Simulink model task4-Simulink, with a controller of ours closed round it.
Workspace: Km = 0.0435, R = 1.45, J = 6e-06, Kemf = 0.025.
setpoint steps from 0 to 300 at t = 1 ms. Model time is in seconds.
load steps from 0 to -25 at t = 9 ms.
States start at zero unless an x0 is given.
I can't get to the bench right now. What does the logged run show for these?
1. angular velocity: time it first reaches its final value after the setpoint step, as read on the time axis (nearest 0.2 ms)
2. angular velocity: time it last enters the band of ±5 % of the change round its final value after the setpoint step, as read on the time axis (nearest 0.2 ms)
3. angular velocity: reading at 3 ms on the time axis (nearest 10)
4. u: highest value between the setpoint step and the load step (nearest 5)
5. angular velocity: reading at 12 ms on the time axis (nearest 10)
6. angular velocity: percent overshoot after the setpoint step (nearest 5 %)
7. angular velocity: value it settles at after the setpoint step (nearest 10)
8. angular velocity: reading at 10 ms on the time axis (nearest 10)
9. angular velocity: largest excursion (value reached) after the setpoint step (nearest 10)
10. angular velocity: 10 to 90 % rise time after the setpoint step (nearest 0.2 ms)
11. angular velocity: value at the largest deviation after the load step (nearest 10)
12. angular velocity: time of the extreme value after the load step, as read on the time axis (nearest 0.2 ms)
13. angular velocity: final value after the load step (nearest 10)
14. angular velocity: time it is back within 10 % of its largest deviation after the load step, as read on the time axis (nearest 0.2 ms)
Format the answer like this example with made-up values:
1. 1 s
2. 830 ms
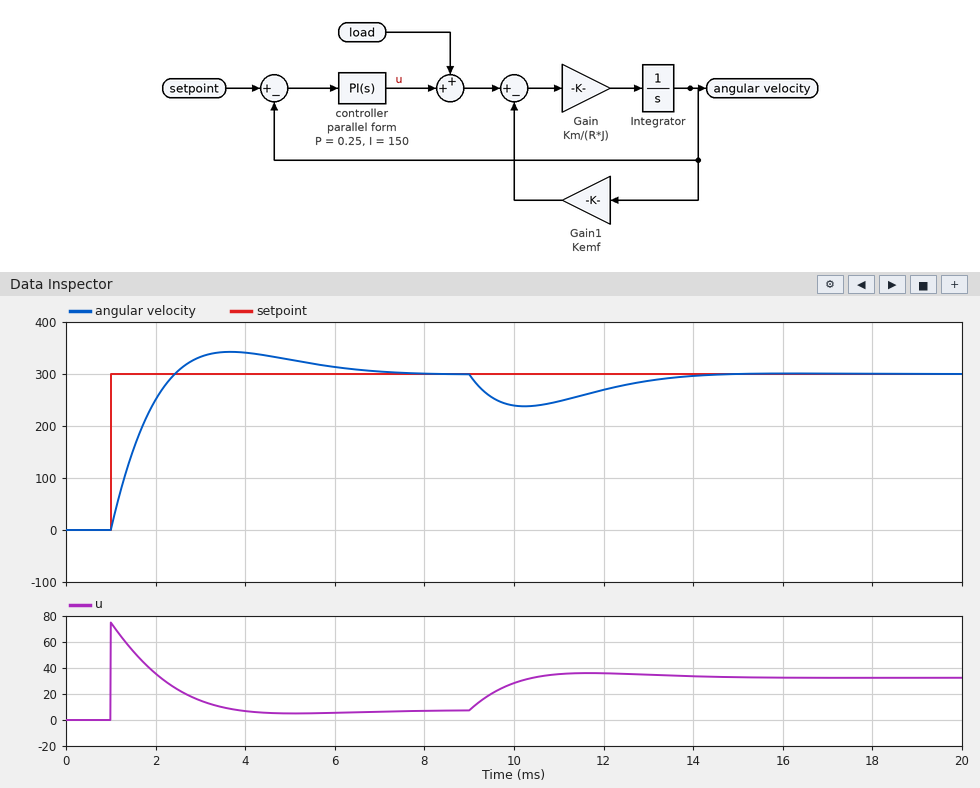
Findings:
1. 2.4 ms
2. 5.8 ms
3. 330
4. 75
5. 270
6. 15 %
7. 300
8. 240
9. 340
10. 1.0 ms
11. 240
12. 10.2 ms
13. 300
14. 13.6 ms
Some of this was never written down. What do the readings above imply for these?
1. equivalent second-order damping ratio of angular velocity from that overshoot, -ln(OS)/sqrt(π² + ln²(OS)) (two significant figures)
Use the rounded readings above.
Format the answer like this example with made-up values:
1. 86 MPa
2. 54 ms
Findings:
1. 0.52
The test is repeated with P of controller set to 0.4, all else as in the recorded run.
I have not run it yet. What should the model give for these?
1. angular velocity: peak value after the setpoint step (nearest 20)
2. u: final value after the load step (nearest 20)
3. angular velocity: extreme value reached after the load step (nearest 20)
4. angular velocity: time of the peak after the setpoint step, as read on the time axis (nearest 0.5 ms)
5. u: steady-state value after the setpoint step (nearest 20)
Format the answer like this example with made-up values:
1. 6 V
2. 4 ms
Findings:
1. 320
2. 40
3. 260
4. 3.5 ms
5. 0
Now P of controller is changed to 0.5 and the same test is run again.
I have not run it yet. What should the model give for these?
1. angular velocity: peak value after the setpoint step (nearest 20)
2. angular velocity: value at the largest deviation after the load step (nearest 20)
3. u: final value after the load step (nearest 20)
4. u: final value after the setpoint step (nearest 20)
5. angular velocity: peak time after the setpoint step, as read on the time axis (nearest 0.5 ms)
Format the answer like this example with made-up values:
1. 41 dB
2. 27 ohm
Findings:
1. 320
2. 260
3. 40
4. 0
5. 3.0 ms
